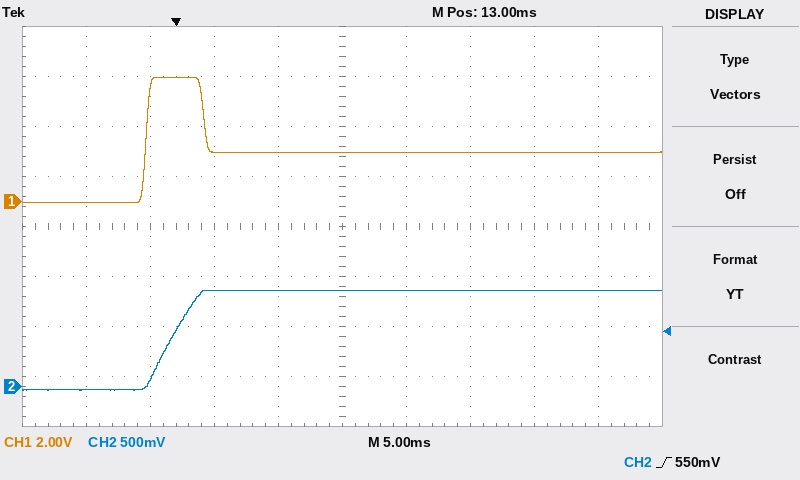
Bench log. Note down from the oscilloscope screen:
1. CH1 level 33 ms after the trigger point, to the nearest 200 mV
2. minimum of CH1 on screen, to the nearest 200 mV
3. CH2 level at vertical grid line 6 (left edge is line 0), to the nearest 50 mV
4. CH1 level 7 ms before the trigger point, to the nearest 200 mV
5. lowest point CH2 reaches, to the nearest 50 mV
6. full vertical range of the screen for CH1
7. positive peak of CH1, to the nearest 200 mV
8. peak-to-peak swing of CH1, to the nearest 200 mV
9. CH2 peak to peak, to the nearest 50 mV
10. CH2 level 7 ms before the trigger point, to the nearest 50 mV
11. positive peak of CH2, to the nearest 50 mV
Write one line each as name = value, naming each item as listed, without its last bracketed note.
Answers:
CH1 level 33 ms after the trigger point, to the nearest 200 mV = 2.0 V
minimum of CH1 on screen, to the nearest 200 mV = 0.0 V
CH2 level at vertical grid line 6 (left edge is line 0), to the nearest 50 mV = 950 mV
CH1 level 7 ms before the trigger point, to the nearest 200 mV = 0.0 V
lowest point CH2 reaches, to the nearest 50 mV = -50 mV
full vertical range of the screen for CH1 = 16 V
positive peak of CH1, to the nearest 200 mV = 5.0 V
peak-to-peak swing of CH1, to the nearest 200 mV = 5.0 V
CH2 peak to peak, to the nearest 50 mV = 1.00 V
CH2 level 7 ms before the trigger point, to the nearest 50 mV = -50 mV
positive peak of CH2, to the nearest 50 mV = 950 mV
